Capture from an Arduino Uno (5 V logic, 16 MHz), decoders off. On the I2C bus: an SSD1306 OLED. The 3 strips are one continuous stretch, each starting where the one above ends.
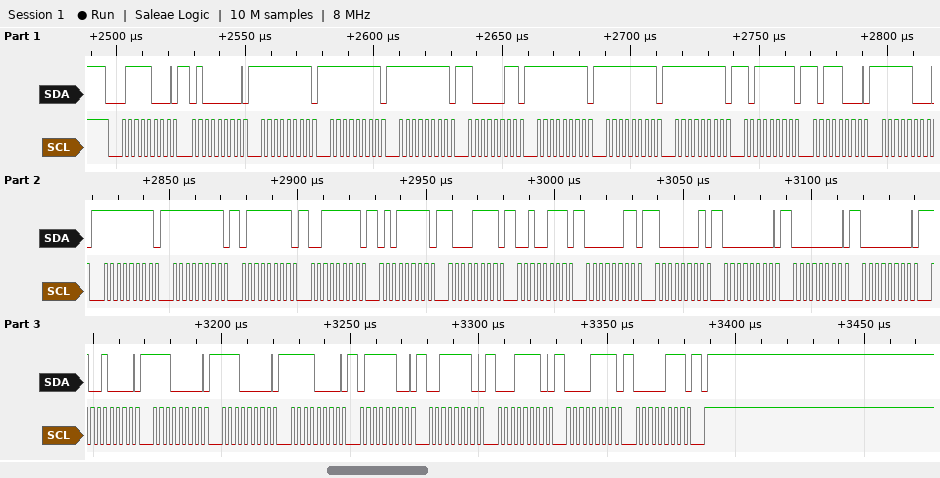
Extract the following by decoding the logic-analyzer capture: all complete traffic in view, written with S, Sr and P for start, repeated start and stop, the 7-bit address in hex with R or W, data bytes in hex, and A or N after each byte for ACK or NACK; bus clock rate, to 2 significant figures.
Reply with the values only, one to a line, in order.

S 3CW A 40 A FF A FF A FF A 83 A FF A FF A FF A BF A B8 A F8 A FF A FF A 7F A 3F A 5F A 8F A 27 A 03 A 81 A 00 A 00 A 00 A 90 A E0 A E0 A F0 A 7C A 3E A 1E A 0F A 07 A P
400 kHz
